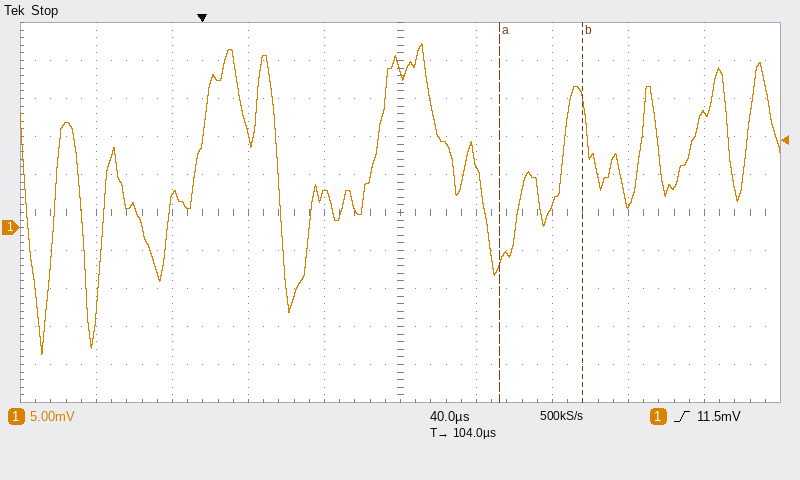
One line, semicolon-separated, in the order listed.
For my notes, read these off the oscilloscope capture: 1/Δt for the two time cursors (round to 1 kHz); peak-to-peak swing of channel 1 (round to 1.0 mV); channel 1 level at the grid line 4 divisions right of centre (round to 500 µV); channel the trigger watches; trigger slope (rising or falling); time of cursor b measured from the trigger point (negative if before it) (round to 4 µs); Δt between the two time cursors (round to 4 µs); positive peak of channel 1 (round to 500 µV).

23 kHz; 41.0 mV; 15.0 mV; channel 1; rising; +200 µs; 44 µs; 24.0 mV
